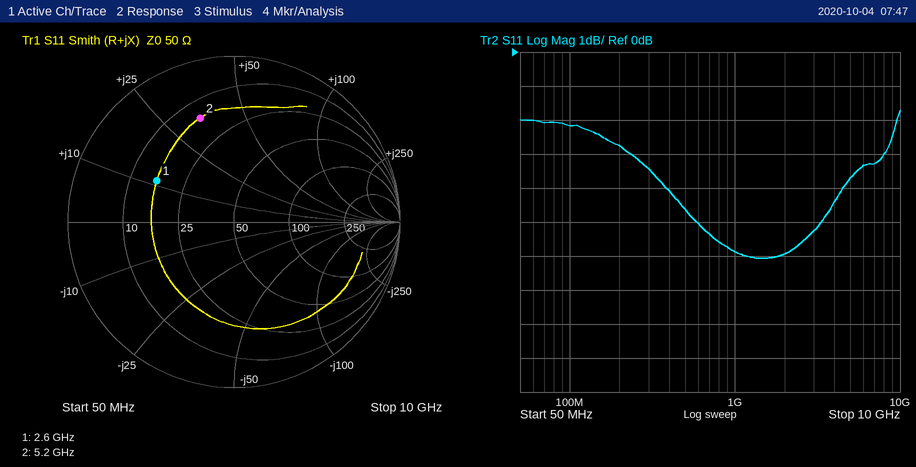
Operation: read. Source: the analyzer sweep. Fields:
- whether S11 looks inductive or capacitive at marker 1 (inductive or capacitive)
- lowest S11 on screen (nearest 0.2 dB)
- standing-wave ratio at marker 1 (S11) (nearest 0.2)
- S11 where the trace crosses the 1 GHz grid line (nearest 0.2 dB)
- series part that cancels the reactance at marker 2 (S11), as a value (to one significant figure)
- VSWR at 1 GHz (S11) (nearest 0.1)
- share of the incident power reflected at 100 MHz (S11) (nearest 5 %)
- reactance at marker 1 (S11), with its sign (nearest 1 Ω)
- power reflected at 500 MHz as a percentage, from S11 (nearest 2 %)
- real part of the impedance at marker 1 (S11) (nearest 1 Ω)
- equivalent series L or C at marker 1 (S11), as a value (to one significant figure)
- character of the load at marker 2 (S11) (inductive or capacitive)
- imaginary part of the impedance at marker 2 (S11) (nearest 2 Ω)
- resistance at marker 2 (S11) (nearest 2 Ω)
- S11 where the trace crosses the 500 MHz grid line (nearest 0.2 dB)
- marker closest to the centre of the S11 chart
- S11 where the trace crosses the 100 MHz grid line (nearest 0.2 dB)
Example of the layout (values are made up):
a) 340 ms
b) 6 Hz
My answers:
a) inductive
b) -6.0 dB
c) 3.2
d) -5.8 dB
e) 900 fF
f) 3.1
g) 60 %
h) +11 Ω
i) 34 %
j) 16 Ω
k) 700 pH
l) inductive
m) +34 Ω
n) 16 Ω
o) -4.6 dB
p) marker 1
q) -2.2 dB
